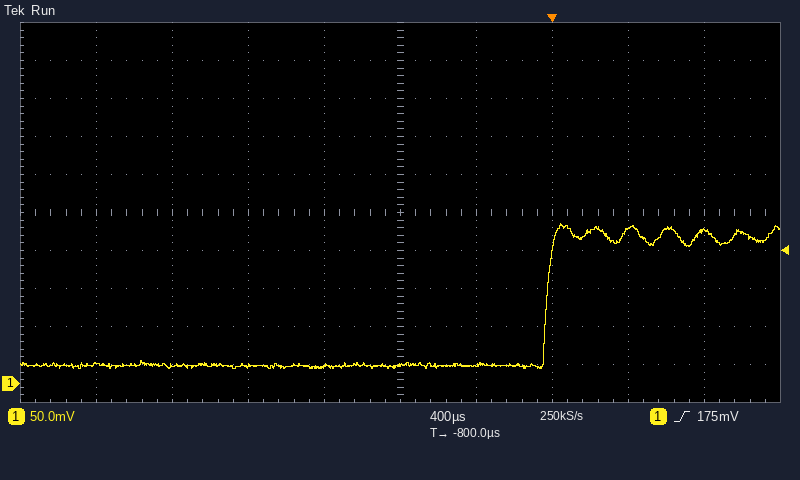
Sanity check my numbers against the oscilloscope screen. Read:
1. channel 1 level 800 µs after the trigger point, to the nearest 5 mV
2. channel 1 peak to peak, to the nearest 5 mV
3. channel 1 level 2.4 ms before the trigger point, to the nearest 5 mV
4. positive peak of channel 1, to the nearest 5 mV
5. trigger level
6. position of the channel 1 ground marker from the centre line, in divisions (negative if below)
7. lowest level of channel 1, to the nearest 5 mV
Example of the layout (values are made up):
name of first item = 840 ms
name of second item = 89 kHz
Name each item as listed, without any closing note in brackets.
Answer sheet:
channel 1 level 800 µs after the trigger point, to the nearest 5 mV = 200 mV
channel 1 peak to peak, to the nearest 5 mV = 190 mV
channel 1 level 2.4 ms before the trigger point, to the nearest 5 mV = 25 mV
positive peak of channel 1, to the nearest 5 mV = 210 mV
trigger level = 175 mV
position of the channel 1 ground marker from the centre line, in divisions = -4.5 div
lowest level of channel 1, to the nearest 5 mV = 20 mV
